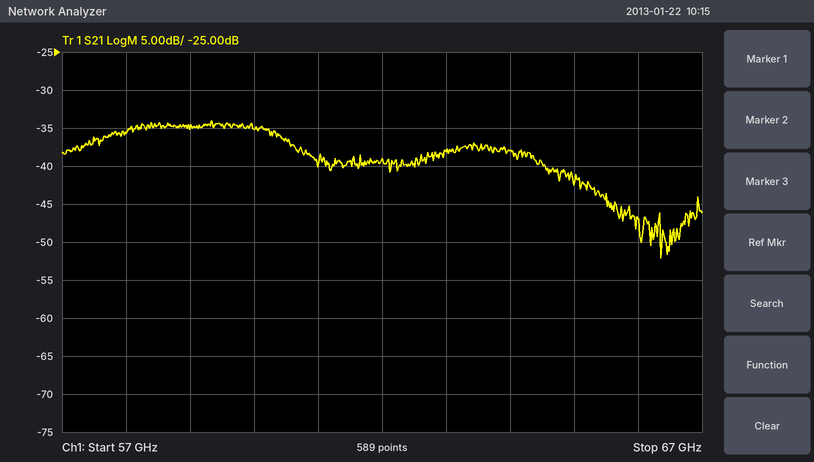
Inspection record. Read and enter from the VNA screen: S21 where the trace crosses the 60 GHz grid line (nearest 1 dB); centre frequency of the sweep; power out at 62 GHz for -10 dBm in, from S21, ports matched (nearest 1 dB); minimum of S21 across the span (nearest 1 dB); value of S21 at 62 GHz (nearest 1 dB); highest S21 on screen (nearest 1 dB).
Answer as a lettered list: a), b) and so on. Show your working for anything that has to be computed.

a) -35 dB
b) 62 GHz
c) -10 dBm + (-39 dB) = -49 dBm
d) -52 dB
e) -39 dB
f) -34 dB
